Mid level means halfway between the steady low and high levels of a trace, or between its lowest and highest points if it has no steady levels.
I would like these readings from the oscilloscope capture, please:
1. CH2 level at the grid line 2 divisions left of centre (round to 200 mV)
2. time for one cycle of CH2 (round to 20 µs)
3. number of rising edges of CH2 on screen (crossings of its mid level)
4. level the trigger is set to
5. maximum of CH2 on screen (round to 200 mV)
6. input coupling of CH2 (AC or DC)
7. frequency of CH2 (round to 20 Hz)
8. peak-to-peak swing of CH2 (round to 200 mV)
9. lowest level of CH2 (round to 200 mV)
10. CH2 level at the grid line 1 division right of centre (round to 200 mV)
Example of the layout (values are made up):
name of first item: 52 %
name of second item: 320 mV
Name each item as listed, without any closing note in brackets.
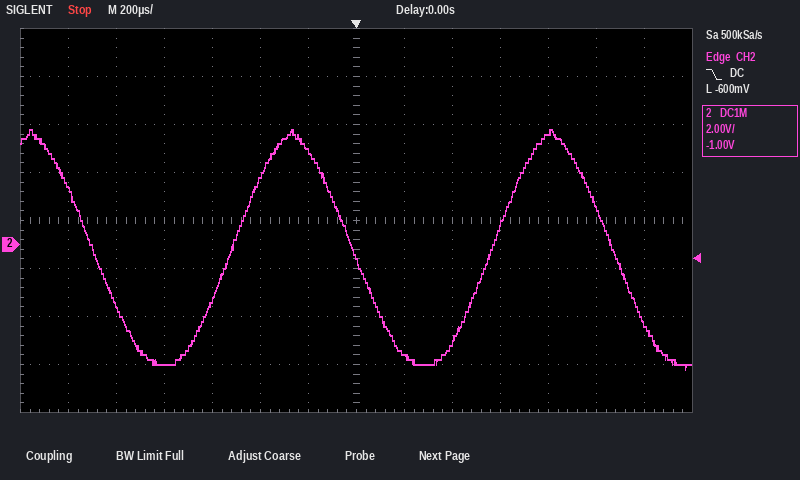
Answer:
CH2 level at the grid line 2 divisions left of centre: 2.8 V
time for one cycle of CH2: 1.08 ms
number of rising edges of CH2 on screen: 2
level the trigger is set to: -600 mV
maximum of CH2 on screen: 4.8 V
input coupling of CH2: DC
frequency of CH2: 920 Hz
peak-to-peak swing of CH2: 10.0 V
lowest level of CH2: -5.2 V
CH2 level at the grid line 1 division right of centre: -4.6 V
